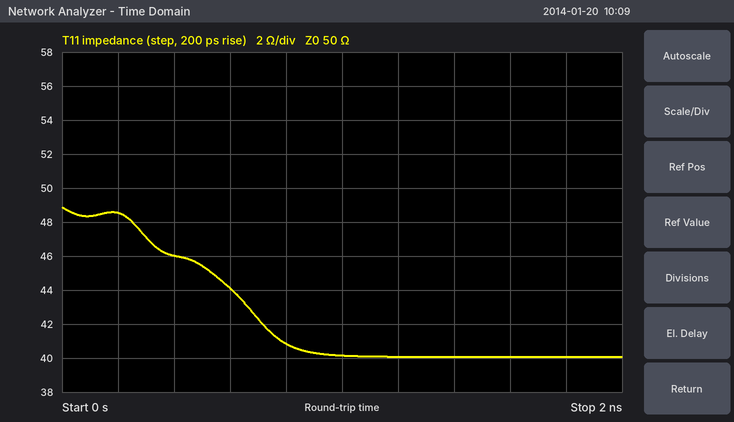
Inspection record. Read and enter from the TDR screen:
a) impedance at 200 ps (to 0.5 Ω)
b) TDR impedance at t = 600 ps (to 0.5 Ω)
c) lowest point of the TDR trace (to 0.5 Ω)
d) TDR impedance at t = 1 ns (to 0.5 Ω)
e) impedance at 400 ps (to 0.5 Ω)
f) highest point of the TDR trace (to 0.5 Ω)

48.5 Ω
44.0 Ω
40.0 Ω
40.0 Ω
46.0 Ω
49.0 Ω
